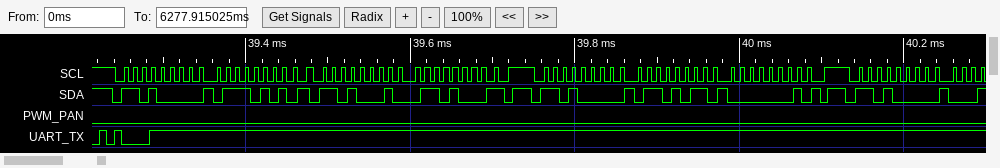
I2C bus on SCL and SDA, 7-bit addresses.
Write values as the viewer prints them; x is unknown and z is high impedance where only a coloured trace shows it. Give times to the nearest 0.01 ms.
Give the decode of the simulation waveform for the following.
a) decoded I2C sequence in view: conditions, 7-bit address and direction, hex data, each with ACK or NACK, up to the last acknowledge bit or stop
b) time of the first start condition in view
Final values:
start, address 68 write ACK, 75 ACK, repeated start, address 68 read ACK, 68 NACK, stop, start, address 68 write ACK, 6B ACK, 01 ACK, stop, start, address 68 write ACK
39.24 ms
